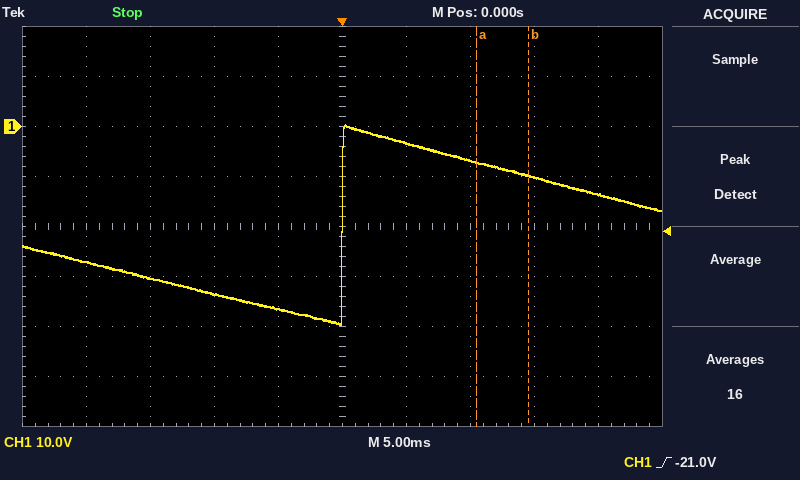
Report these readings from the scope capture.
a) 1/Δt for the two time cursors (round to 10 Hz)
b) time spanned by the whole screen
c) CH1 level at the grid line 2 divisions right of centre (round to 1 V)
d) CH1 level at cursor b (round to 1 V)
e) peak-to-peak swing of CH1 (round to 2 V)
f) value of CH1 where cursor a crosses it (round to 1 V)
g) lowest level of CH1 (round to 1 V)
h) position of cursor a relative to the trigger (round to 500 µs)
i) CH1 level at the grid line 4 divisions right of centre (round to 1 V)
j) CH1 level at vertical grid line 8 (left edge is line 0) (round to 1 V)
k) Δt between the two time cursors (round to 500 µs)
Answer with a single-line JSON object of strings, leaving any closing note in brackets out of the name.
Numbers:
{"1/Δt for the two time cursors": "250 Hz", "time spanned by the whole screen": "50 ms", "CH1 level at the grid line 2 divisions right of centre": "-7 V", "CH1 level at cursor b": "-10 V", "peak-to-peak swing of CH1": "40 V", "value of CH1 where cursor a crosses it": "-7 V", "lowest level of CH1": "-40 V", "position of cursor a relative to the trigger": "+10.5 ms", "CH1 level at the grid line 4 divisions right of centre": "-14 V", "CH1 level at vertical grid line 8 (left edge is line 0)": "-10 V", "Δt between the two time cursors": "4.0 ms"}
